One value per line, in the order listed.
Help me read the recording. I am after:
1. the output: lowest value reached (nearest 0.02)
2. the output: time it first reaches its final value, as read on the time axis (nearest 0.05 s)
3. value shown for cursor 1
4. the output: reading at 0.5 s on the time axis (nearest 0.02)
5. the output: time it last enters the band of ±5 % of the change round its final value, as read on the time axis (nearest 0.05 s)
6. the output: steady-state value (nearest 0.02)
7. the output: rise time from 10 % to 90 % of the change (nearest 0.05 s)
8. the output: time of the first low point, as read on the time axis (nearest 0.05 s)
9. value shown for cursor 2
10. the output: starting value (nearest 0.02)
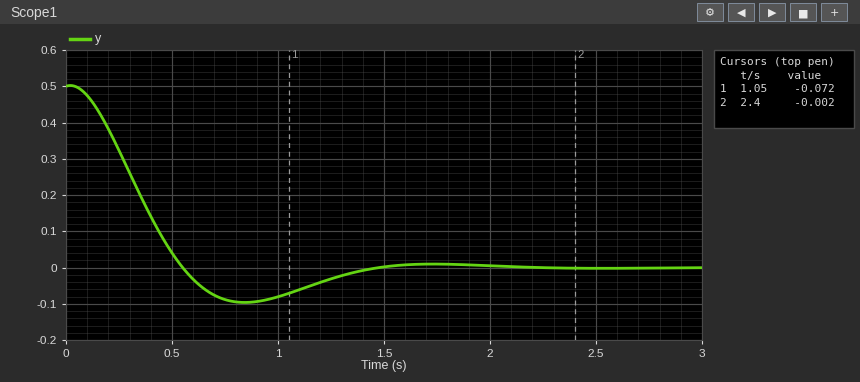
-0.10
0.55 s
-0.072
0.04
1.30 s
0.00
0.35 s
0.85 s
-0.002
0.50
